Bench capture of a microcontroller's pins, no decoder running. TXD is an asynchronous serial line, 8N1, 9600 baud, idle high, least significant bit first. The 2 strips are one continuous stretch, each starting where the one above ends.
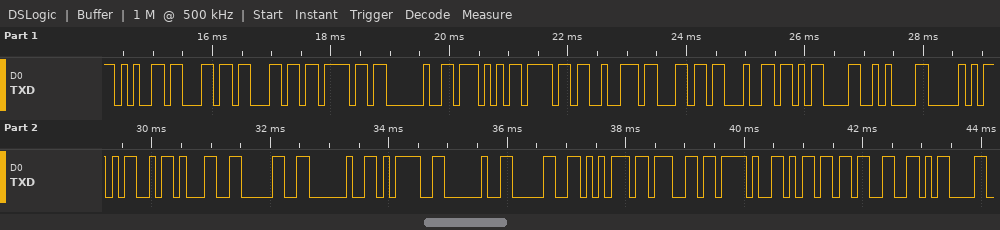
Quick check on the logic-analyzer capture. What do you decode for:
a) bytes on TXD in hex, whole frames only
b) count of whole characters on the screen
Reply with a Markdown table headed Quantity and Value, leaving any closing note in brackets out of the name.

| Quantity | Value |
|---|---|
| bytes on TXD in hex, whole frames only | 65 6C 6C 6F 20 57 6F 72 6C 64 0D 0A 50 4D 31 30 20 3D 20 30 75 67 2F 6D 33 0D |
| count of whole characters on the screen | 26 |
